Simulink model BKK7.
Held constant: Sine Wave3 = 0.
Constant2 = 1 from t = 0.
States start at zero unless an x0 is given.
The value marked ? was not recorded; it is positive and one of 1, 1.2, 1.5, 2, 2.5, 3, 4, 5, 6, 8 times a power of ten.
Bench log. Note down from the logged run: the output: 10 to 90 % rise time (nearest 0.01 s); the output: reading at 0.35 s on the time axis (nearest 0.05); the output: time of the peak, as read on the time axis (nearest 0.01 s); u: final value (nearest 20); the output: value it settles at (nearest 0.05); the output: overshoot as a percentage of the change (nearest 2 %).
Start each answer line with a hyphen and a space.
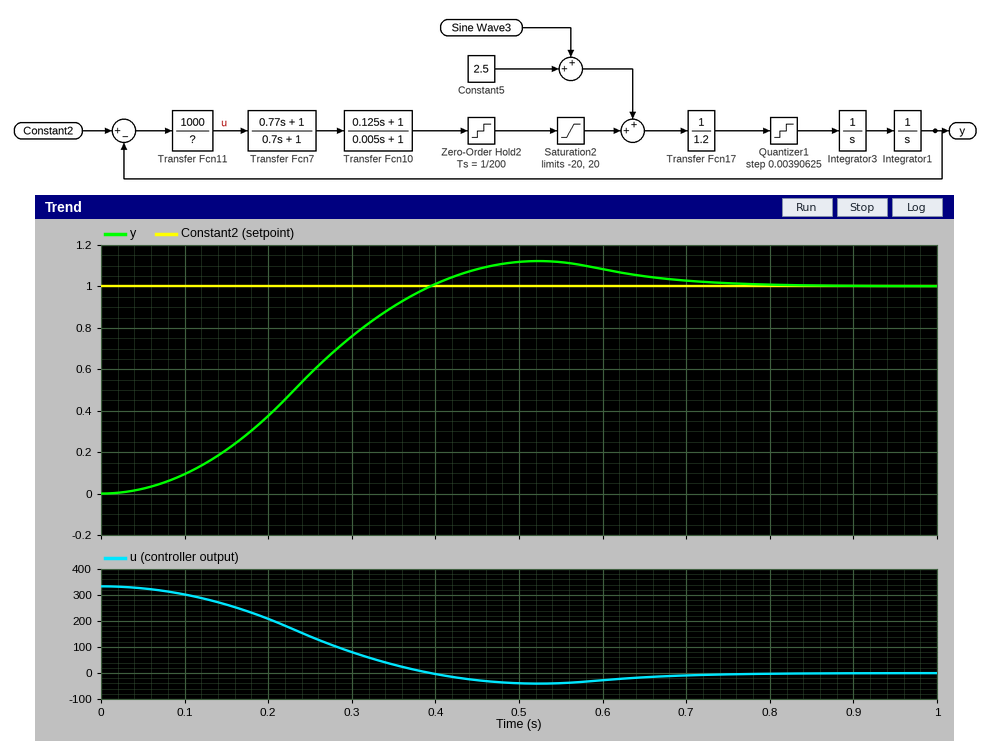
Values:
- 0.25 s
- 0.90
- 0.52 s
- 0
- 1.00
- 12 %
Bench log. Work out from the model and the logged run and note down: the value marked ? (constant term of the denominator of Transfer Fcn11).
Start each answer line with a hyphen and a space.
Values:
- 3
